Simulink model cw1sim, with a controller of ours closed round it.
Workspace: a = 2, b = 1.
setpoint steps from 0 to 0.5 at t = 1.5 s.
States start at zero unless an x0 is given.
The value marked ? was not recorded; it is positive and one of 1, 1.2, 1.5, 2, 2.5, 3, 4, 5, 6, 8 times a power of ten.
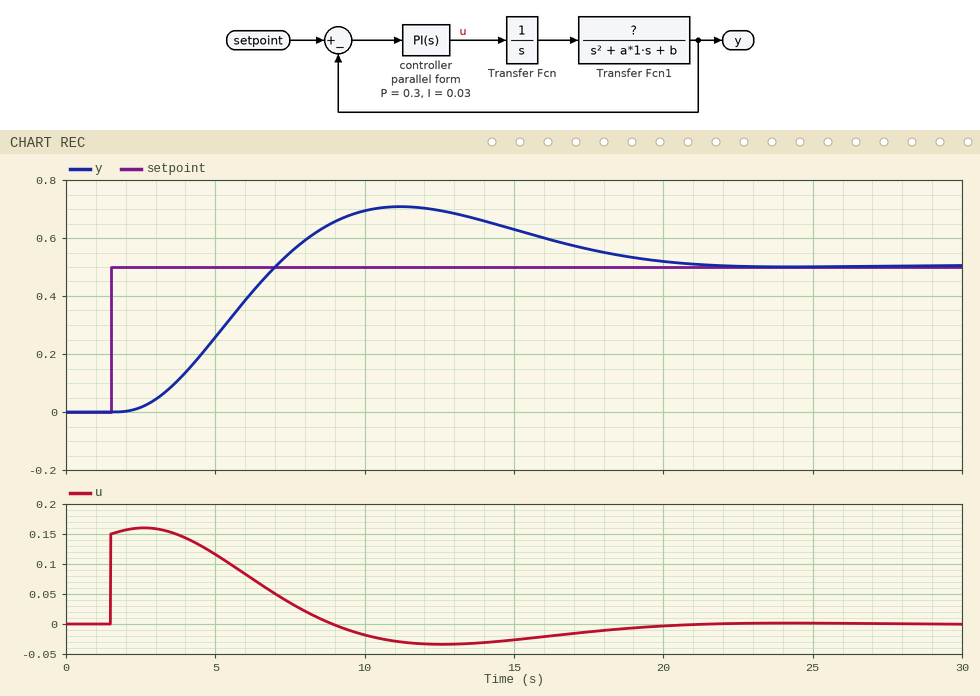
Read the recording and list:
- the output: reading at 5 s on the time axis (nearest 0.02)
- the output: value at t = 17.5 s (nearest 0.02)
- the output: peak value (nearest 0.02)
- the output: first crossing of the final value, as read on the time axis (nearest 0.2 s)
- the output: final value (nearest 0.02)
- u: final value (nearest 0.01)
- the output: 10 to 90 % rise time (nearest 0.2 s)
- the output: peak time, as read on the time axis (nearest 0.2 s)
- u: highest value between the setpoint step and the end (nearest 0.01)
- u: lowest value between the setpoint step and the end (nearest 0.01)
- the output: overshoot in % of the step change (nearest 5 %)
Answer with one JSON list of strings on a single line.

["0.26", "0.56", "0.70", "7.0 s", "0.50", "0.00", "3.4 s", "11.2 s", "0.16", "-0.03", "40 %"]
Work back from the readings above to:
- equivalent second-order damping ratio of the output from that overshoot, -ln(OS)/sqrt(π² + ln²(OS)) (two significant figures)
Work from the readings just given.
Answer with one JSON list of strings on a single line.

["0.28"]
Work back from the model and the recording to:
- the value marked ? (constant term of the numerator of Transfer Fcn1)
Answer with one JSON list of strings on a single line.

["1"]
